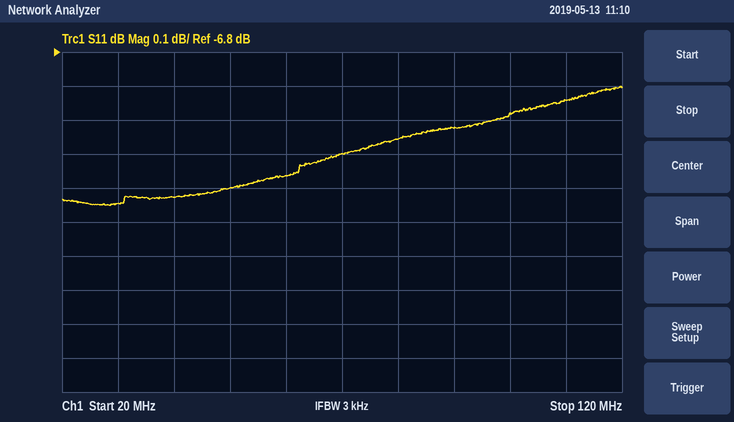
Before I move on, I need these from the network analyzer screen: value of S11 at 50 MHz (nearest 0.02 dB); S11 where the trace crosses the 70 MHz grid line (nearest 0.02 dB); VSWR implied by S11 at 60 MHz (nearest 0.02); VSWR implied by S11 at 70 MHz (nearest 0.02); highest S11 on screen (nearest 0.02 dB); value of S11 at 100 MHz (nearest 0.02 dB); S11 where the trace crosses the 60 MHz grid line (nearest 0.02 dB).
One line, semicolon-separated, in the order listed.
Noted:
-7.20 dB; -7.10 dB; 2.56; 2.58; -6.90 dB; -6.98 dB; -7.16 dB
